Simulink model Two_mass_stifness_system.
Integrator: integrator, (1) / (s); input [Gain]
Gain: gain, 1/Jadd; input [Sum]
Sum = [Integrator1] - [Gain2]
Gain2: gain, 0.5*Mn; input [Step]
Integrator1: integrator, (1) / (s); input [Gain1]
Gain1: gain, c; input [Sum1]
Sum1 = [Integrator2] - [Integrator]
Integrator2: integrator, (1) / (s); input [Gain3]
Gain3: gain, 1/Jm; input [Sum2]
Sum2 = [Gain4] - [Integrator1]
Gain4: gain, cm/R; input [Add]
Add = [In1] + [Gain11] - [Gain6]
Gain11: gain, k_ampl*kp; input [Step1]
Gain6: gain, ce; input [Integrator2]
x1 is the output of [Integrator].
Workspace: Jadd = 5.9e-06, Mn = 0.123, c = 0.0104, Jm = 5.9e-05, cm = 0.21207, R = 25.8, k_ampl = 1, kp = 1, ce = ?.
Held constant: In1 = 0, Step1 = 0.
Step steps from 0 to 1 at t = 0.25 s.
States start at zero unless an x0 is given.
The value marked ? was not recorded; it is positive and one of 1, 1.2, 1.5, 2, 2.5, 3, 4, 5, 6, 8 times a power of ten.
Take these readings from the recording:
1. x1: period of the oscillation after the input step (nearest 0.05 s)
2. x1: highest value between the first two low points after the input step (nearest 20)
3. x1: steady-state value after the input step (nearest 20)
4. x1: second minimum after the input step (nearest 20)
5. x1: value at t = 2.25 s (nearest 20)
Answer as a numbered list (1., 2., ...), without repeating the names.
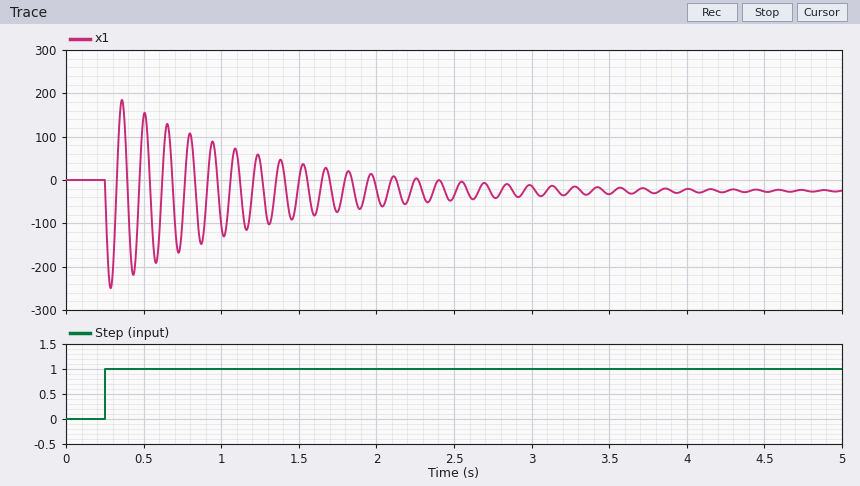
1. 0.15 s
2. 180
3. -20
4. -220
5. 0
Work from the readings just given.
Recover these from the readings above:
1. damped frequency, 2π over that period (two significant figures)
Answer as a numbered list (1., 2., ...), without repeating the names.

1. 42 rad/s
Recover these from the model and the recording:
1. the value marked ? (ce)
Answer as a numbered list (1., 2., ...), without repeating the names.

1. 0.3
